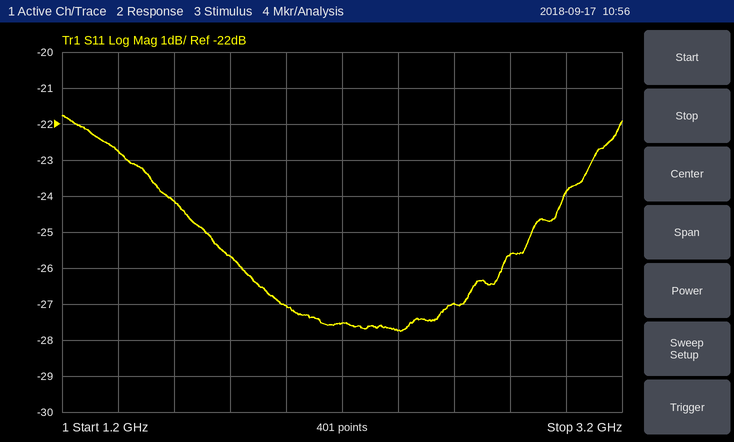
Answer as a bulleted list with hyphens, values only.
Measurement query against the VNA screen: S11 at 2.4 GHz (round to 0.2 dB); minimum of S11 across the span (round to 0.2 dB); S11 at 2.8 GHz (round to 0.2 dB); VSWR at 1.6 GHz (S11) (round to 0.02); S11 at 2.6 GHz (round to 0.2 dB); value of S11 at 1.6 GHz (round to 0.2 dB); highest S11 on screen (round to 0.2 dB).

- -27.8 dB
- -27.8 dB
- -25.6 dB
- 1.14
- -27.0 dB
- -24.2 dB
- -21.8 dB
